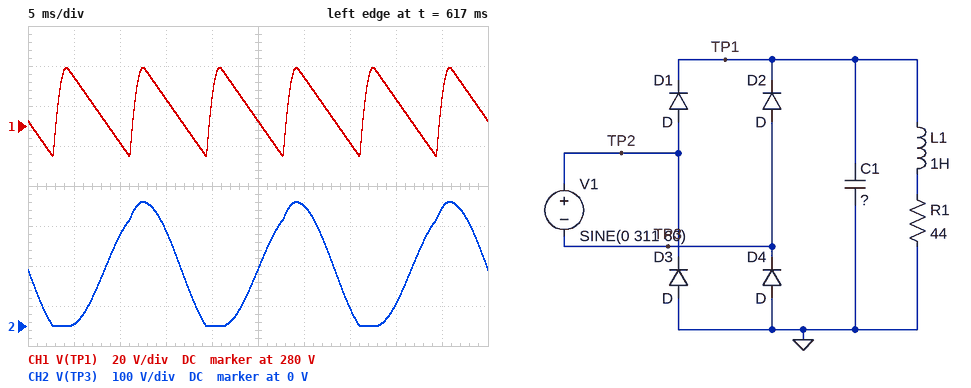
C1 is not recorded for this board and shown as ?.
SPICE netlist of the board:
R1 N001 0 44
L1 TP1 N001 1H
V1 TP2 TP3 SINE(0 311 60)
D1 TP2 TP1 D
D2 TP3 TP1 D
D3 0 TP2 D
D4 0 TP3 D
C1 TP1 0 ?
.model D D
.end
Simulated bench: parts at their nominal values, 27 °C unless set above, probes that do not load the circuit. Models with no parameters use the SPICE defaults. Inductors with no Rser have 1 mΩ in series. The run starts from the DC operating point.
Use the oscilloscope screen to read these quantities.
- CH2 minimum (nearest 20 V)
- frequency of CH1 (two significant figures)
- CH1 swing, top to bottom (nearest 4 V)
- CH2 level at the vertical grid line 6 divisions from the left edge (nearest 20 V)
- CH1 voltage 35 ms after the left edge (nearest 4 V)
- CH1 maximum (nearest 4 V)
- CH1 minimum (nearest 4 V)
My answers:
0 V
120 Hz
44 V
300 V
272 V
308 V
264 V
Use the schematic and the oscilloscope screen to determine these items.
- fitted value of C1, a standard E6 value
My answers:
1 mF
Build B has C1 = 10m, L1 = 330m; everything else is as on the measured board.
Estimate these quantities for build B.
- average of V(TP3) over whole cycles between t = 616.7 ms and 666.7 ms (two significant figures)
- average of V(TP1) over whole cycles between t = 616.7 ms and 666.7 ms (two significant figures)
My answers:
150 V
310 V
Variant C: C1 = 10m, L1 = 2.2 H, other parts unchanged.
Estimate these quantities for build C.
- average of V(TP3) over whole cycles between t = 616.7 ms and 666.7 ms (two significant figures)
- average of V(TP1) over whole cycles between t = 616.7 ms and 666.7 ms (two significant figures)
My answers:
150 V
310 V
